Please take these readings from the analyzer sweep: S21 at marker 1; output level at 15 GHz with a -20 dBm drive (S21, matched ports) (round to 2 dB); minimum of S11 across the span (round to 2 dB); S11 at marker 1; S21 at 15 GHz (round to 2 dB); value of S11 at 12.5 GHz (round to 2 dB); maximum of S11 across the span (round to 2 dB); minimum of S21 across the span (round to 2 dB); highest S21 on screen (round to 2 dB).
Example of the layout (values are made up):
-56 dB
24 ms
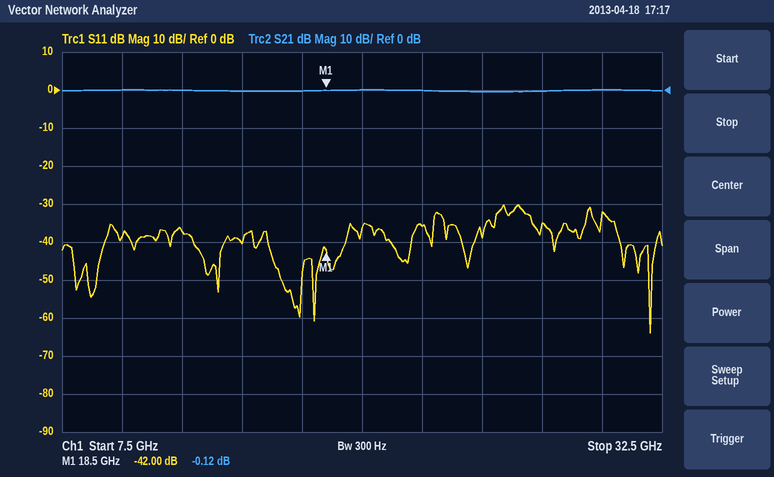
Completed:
-0.12 dB
-20 dBm
-64 dB
-42.00 dB
0 dB
-38 dB
-30 dB
0 dB
0 dB
